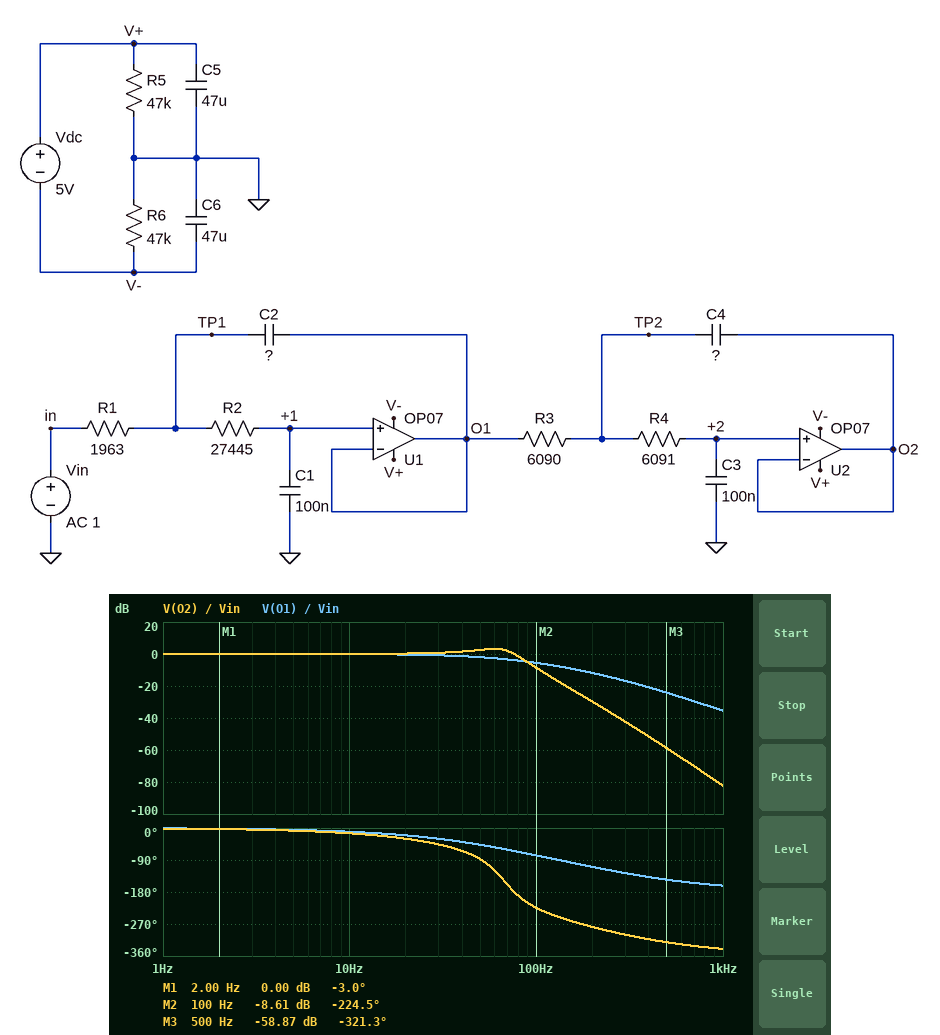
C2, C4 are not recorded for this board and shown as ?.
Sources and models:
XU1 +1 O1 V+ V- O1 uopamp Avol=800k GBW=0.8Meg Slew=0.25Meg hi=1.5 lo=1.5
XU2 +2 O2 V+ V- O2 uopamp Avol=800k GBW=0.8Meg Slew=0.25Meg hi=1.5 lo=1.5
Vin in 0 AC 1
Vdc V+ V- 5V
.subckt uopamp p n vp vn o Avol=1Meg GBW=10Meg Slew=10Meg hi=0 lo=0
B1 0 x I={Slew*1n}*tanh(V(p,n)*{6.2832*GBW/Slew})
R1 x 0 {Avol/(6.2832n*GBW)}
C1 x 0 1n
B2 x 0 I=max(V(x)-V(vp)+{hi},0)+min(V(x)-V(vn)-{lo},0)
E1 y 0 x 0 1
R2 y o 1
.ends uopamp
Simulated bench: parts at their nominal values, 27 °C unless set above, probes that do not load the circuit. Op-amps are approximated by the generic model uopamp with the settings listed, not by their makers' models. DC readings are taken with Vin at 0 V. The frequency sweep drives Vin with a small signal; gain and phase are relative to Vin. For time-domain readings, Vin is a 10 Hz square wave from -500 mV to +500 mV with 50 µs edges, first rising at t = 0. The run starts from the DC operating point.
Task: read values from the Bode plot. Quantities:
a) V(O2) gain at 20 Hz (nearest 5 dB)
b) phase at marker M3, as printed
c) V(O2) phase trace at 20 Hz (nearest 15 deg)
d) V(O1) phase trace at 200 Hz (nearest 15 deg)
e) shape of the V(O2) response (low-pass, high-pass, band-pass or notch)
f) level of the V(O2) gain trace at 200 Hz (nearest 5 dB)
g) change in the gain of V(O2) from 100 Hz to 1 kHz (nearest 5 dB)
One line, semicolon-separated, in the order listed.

0 dB; -321.3 deg; -30 deg; -105 deg; low-pass; -30 dB; -75 dB
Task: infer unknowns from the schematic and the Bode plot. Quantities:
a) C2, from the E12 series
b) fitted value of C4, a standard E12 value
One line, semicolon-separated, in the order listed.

270 nF; 1.5 µF
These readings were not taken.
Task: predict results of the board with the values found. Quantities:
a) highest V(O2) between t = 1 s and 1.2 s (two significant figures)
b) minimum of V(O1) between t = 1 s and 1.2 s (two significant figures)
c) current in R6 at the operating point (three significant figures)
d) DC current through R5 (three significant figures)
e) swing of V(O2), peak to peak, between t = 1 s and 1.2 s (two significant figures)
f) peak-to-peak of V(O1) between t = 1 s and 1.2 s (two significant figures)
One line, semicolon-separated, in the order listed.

760 mV; -500 mV; 53.2 µA; 53.2 µA; 1.5 V; 1.0 V
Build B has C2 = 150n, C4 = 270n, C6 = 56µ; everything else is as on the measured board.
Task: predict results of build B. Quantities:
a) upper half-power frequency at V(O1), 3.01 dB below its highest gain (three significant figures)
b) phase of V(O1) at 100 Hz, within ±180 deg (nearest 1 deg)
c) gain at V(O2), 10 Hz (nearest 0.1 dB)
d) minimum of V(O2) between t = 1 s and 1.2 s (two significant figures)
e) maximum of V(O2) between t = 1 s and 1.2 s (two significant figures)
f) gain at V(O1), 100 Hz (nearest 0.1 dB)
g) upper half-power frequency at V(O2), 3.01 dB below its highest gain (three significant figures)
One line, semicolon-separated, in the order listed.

59.6 Hz; -70 deg; -0.1 dB; -500 mV; 500 mV; -5.9 dB; 63.1 Hz
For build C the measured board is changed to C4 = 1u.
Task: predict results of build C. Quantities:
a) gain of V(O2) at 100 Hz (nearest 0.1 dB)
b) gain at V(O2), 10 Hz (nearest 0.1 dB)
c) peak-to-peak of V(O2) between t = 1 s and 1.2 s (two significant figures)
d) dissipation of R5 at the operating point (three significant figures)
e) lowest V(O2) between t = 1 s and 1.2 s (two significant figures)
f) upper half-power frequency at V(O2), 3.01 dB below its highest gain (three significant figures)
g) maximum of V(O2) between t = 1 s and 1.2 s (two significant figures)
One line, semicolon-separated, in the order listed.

-4.6 dB; 0 dB; 1.3 V; 133 µW; -660 mV; 90.3 Hz; 660 mV
